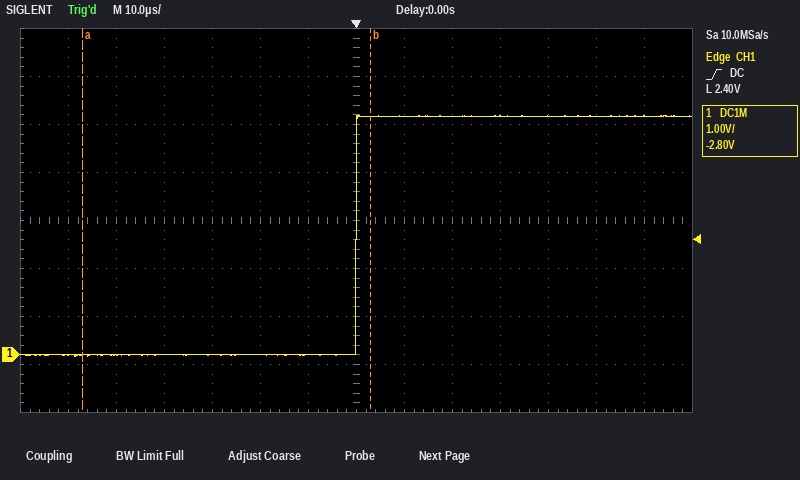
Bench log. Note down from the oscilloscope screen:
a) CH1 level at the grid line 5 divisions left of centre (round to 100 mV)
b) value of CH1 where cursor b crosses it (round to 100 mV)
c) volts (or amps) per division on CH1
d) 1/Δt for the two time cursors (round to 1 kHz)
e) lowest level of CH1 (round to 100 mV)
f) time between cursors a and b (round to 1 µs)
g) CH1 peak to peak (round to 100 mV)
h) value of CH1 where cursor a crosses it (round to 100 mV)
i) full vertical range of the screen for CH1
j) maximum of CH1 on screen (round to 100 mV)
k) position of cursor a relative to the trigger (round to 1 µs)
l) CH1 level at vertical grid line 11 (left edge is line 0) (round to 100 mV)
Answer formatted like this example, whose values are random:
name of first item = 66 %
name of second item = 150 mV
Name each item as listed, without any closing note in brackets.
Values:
CH1 level at the grid line 5 divisions left of centre = 0.0 V
value of CH1 where cursor b crosses it = 5.0 V
volts (or amps) per division on CH1 = 1 V
1/Δt for the two time cursors = 17 kHz
lowest level of CH1 = 0.0 V
time between cursors a and b = 60 µs
CH1 peak to peak = 5.0 V
value of CH1 where cursor a crosses it = 0.0 V
full vertical range of the screen for CH1 = 8 V
maximum of CH1 on screen = 5.0 V
position of cursor a relative to the trigger = -57 µs
CH1 level at vertical grid line 11 (left edge is line 0) = 5.0 V
